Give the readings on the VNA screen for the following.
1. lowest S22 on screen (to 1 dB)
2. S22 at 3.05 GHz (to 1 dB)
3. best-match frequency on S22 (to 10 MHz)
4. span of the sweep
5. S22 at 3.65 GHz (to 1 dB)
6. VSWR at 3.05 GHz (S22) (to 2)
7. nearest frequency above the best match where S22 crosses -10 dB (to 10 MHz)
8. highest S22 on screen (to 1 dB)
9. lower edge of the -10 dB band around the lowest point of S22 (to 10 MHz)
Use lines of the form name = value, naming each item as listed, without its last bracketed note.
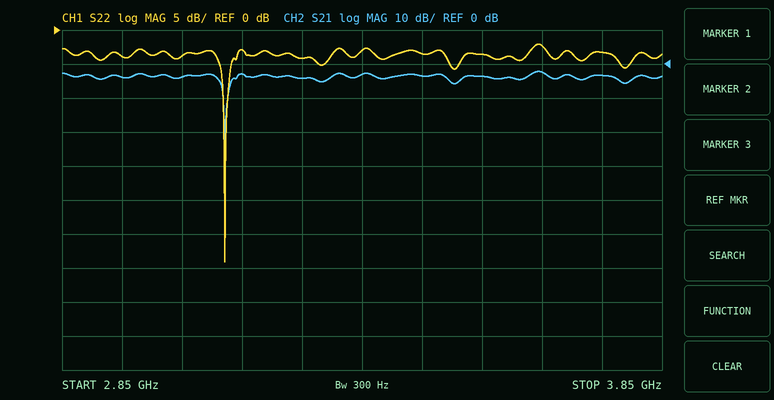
lowest S22 on screen = -34 dB
S22 at 3.05 GHz = -4 dB
best-match frequency on S22 = 3.12 GHz
span of the sweep = 1 GHz
S22 at 3.65 GHz = -2 dB
VSWR at 3.05 GHz (S22) = 4
nearest frequency above the best match where S22 crosses -10 dB = 3.13 GHz
highest S22 on screen = -2 dB
lower edge of the -10 dB band around the lowest point of S22 = 3.12 GHz
